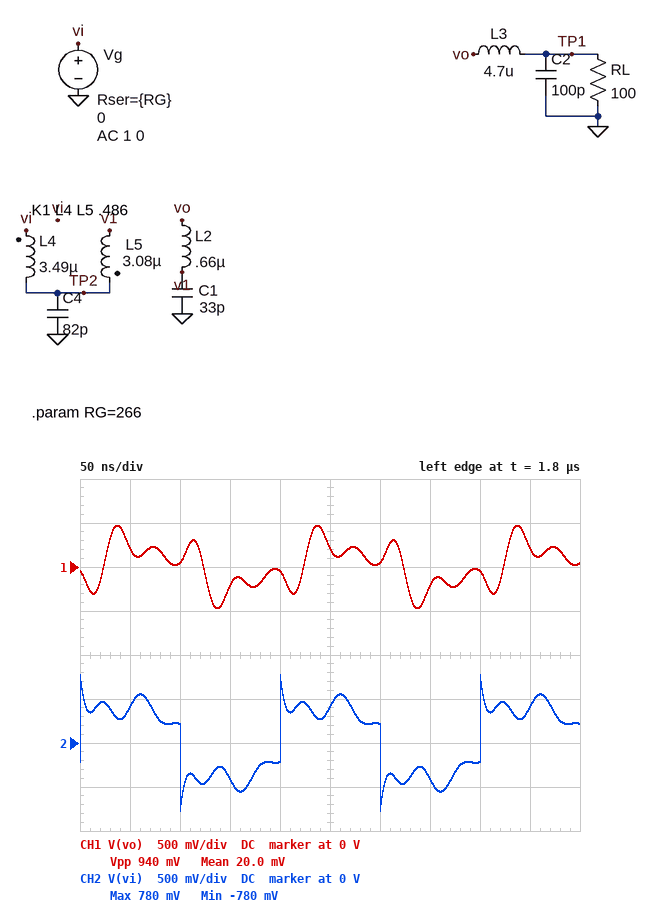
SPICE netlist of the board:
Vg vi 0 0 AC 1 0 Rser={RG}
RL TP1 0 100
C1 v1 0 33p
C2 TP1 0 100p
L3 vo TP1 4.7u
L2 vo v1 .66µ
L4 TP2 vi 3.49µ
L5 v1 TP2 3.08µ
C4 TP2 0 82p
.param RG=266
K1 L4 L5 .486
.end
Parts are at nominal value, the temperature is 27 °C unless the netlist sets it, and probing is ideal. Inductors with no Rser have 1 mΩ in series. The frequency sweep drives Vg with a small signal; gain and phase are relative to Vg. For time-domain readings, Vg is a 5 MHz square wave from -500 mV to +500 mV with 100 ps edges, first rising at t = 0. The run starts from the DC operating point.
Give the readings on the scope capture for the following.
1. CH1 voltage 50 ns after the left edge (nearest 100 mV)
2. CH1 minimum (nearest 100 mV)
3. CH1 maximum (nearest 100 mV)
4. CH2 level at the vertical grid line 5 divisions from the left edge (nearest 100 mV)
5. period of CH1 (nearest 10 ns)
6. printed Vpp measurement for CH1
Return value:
200 mV
-500 mV
500 mV
400 mV
200 ns
940 mV
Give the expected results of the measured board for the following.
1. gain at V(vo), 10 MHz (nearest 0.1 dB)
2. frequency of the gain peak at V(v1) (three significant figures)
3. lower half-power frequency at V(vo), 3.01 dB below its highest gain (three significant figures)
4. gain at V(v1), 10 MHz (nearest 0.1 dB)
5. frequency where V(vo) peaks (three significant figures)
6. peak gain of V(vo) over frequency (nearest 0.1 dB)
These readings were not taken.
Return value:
-2.6 dB
25.3 MHz
21.8 MHz
-1.3 dB
25.3 MHz
2.3 dB
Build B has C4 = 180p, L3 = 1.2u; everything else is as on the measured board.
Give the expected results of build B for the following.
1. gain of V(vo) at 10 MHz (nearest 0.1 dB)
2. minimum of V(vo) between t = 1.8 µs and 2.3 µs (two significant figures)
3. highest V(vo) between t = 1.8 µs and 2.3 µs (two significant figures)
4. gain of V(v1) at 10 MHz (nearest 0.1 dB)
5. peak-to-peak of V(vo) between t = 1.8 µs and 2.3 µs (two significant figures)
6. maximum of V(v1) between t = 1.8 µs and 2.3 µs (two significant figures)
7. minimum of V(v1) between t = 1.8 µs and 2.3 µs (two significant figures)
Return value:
-12.3 dB
-240 mV
240 mV
-10.0 dB
480 mV
280 mV
-280 mV
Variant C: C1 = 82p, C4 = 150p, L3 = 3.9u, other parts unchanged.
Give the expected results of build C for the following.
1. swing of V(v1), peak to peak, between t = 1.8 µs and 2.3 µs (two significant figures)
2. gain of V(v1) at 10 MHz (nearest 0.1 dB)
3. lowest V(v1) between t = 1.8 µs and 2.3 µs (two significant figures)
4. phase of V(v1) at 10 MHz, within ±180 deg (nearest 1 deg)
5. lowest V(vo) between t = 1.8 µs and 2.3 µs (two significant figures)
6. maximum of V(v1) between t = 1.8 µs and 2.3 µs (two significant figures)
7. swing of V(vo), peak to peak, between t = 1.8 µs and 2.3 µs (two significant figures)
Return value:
830 mV
-4.0 dB
-410 mV
-124 deg
-340 mV
410 mV
690 mV
